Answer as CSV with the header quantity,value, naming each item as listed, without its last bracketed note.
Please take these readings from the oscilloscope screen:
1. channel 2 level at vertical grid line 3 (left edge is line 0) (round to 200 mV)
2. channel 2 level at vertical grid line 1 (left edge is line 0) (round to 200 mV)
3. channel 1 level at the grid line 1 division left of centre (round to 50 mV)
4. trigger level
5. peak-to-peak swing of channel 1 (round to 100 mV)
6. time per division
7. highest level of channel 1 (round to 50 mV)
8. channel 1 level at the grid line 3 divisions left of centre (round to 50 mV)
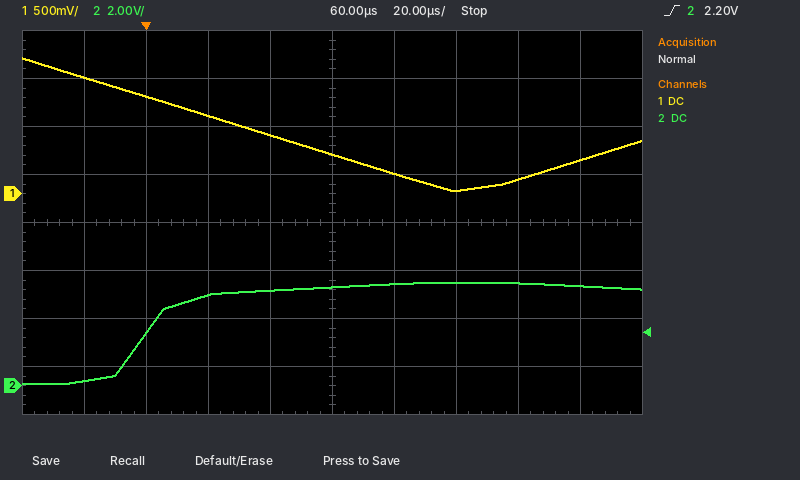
quantity,value
channel 2 level at vertical grid line 3 (left edge is line 0),3.8 V
channel 2 level at vertical grid line 1 (left edge is line 0),200 mV
channel 1 level at the grid line 1 division left of centre,600 mV
trigger level,2.20 V
peak-to-peak swing of channel 1,1.40 V
time per division,20 µs
highest level of channel 1,1.40 V
channel 1 level at the grid line 3 divisions left of centre,1.00 V
